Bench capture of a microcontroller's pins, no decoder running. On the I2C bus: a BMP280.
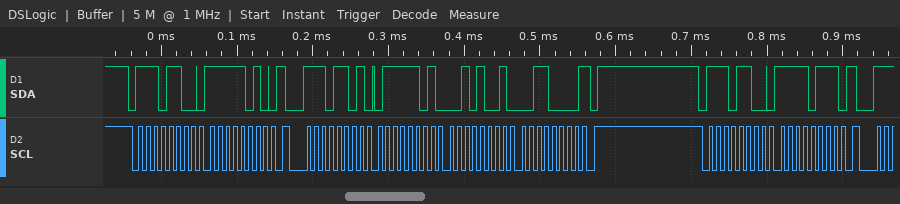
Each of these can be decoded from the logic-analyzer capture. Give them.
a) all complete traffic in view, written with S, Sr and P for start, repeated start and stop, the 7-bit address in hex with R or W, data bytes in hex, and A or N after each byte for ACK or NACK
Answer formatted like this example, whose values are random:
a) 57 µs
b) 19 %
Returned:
a) S 76W A FA A Sr 76R A 7D A 29 A 30 N P S 76W A F7 A
